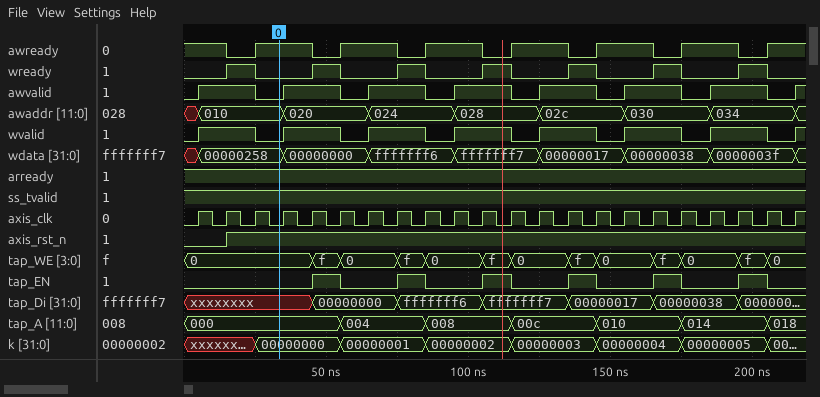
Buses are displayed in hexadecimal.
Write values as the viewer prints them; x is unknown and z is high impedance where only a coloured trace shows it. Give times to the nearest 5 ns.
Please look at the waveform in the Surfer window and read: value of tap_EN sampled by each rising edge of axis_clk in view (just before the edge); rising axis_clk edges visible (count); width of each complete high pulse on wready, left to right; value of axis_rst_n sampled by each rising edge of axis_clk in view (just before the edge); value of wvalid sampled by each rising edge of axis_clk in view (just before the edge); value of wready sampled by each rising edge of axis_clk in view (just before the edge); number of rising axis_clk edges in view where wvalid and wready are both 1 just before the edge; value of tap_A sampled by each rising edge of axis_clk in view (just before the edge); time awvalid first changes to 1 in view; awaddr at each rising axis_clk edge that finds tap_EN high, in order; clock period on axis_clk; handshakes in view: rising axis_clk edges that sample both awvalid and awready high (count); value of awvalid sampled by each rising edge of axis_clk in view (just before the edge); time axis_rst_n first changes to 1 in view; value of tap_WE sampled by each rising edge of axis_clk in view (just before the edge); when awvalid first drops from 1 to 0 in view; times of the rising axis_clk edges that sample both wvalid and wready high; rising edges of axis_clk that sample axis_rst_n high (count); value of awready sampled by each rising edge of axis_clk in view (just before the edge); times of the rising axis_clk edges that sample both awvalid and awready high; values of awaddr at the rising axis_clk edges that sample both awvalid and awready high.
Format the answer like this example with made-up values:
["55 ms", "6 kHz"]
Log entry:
["0 0 0 0 0 1 0 0 1 0 0 1 0 0 1 0 0 1 0 0 1 0", "22", "10 ns, 10 ns, 10 ns, 10 ns, 10 ns, 10 ns, 10 ns", "0 0 1 1 1 1 1 1 1 1 1 1 1 1 1 1 1 1 1 1 1 1", "0 1 1 0 1 1 0 1 1 0 1 1 0 1 1 0 1 1 0 1 1 0", "0 0 1 0 0 1 0 0 1 0 0 1 0 0 1 0 0 1 0 0 1 0", "7", "000, 000, 000, 000, 000, 000, 004, 004, 004, 008, 008, 008, 00c, 00c, 00c, 010, 010, 010, 014, 014, 014, 018", "5 ns", "020, 024, 028, 02c, 030, 034", "10 ns", "7", "0 1 1 0 1 1 0 1 1 0 1 1 0 1 1 0 1 1 0 1 1 0", "15 ns", "0, 0, 0, 0, 0, f, 0, 0, f, 0, 0, f, 0, 0, f, 0, 0, f, 0, 0, f, 0", "25 ns", "25 ns, 55 ns, 85 ns, 115 ns, 145 ns, 175 ns, 205 ns", "20", "1 1 0 1 1 0 1 1 0 1 1 0 1 1 0 1 1 0 1 1 0 1", "15 ns, 45 ns, 75 ns, 105 ns, 135 ns, 165 ns, 195 ns", "010, 020, 024, 028, 02c, 030, 034"]
